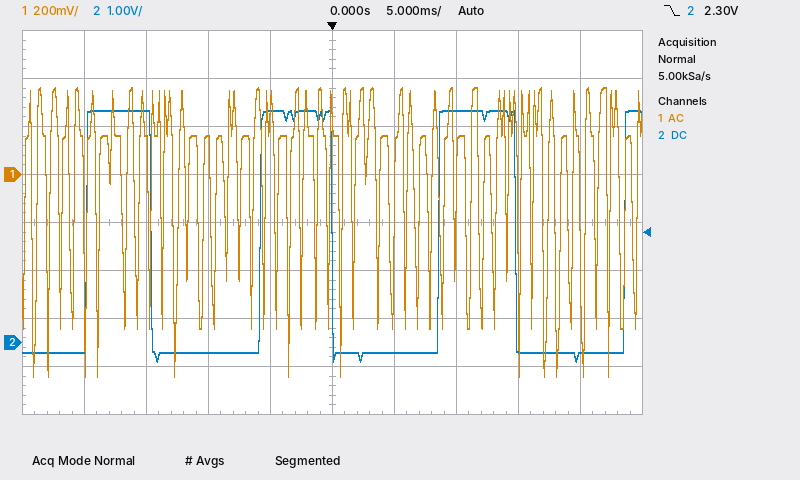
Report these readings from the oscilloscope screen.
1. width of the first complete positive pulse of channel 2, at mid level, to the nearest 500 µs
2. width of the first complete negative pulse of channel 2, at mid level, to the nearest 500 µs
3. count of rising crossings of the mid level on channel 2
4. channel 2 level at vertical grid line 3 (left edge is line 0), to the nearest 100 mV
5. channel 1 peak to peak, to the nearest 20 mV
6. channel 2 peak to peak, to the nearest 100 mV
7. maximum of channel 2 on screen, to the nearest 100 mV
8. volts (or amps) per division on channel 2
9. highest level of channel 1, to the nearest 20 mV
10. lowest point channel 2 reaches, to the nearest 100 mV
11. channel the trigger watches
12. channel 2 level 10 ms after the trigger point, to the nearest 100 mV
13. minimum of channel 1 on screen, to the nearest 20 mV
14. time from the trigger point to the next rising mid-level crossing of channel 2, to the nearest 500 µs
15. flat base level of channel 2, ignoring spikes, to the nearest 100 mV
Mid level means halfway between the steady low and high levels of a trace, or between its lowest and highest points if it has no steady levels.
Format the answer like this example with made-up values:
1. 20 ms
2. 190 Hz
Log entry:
1. 5.0 ms
2. 9.0 ms
3. 4
4. -200 mV
5. 1.20 V
6. 5.2 V
7. 4.8 V
8. 1 V
9. 360 mV
10. -400 mV
11. channel 2
12. 4.8 V
13. -840 mV
14. 8.5 ms
15. -200 mV
